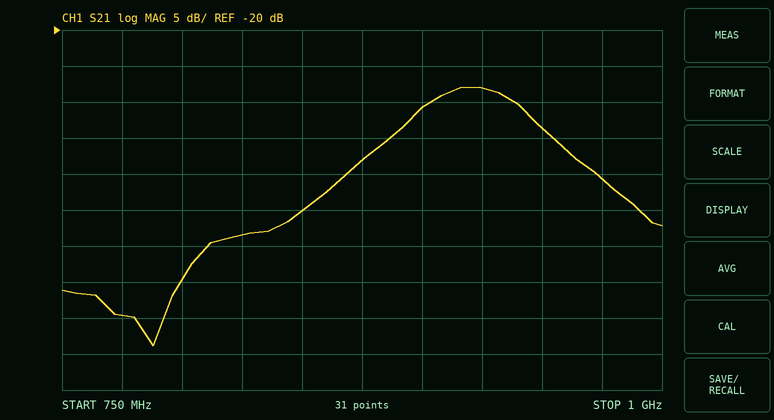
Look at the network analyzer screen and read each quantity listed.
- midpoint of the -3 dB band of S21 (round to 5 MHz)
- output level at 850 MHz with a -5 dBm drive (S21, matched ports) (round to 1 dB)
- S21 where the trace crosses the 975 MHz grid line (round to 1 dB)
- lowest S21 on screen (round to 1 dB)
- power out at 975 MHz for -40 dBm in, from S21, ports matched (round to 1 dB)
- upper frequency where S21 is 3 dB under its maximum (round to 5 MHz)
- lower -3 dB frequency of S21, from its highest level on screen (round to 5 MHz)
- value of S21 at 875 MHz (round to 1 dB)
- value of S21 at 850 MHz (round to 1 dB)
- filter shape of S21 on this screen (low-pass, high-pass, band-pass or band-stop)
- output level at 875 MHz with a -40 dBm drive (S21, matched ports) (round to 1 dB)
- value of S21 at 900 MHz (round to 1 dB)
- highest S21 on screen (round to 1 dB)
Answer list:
920 MHz
-50 dBm
-41 dB
-64 dB
-81 dBm
940 MHz
900 MHz
-38 dB
-45 dB
band-pass
-78 dBm
-31 dB
-28 dB
